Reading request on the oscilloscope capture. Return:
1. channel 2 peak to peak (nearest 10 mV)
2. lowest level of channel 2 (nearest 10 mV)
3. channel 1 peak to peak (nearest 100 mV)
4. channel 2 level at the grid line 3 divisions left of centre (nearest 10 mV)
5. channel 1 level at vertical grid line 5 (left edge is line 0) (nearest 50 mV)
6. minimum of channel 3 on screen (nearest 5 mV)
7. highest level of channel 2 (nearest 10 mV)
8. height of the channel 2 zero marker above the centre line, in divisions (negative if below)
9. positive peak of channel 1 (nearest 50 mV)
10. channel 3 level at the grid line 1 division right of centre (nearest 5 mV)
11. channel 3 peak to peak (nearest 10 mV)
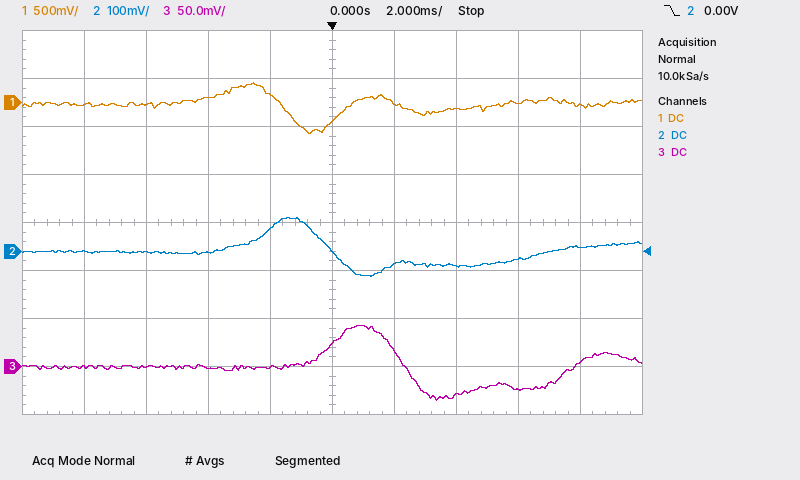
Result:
120 mV
-50 mV
500 mV
0 mV
-200 mV
-35 mV
70 mV
-0.6 div
200 mV
15 mV
80 mV
